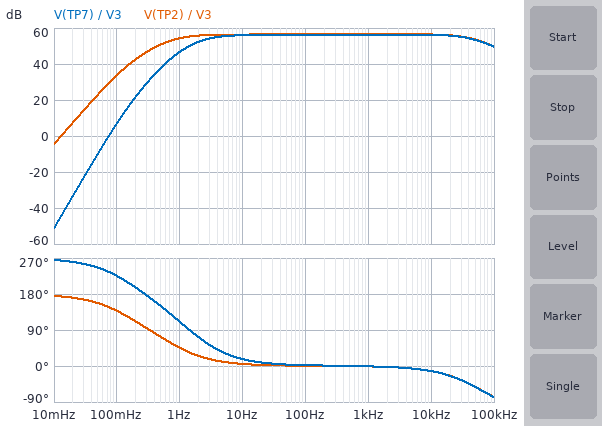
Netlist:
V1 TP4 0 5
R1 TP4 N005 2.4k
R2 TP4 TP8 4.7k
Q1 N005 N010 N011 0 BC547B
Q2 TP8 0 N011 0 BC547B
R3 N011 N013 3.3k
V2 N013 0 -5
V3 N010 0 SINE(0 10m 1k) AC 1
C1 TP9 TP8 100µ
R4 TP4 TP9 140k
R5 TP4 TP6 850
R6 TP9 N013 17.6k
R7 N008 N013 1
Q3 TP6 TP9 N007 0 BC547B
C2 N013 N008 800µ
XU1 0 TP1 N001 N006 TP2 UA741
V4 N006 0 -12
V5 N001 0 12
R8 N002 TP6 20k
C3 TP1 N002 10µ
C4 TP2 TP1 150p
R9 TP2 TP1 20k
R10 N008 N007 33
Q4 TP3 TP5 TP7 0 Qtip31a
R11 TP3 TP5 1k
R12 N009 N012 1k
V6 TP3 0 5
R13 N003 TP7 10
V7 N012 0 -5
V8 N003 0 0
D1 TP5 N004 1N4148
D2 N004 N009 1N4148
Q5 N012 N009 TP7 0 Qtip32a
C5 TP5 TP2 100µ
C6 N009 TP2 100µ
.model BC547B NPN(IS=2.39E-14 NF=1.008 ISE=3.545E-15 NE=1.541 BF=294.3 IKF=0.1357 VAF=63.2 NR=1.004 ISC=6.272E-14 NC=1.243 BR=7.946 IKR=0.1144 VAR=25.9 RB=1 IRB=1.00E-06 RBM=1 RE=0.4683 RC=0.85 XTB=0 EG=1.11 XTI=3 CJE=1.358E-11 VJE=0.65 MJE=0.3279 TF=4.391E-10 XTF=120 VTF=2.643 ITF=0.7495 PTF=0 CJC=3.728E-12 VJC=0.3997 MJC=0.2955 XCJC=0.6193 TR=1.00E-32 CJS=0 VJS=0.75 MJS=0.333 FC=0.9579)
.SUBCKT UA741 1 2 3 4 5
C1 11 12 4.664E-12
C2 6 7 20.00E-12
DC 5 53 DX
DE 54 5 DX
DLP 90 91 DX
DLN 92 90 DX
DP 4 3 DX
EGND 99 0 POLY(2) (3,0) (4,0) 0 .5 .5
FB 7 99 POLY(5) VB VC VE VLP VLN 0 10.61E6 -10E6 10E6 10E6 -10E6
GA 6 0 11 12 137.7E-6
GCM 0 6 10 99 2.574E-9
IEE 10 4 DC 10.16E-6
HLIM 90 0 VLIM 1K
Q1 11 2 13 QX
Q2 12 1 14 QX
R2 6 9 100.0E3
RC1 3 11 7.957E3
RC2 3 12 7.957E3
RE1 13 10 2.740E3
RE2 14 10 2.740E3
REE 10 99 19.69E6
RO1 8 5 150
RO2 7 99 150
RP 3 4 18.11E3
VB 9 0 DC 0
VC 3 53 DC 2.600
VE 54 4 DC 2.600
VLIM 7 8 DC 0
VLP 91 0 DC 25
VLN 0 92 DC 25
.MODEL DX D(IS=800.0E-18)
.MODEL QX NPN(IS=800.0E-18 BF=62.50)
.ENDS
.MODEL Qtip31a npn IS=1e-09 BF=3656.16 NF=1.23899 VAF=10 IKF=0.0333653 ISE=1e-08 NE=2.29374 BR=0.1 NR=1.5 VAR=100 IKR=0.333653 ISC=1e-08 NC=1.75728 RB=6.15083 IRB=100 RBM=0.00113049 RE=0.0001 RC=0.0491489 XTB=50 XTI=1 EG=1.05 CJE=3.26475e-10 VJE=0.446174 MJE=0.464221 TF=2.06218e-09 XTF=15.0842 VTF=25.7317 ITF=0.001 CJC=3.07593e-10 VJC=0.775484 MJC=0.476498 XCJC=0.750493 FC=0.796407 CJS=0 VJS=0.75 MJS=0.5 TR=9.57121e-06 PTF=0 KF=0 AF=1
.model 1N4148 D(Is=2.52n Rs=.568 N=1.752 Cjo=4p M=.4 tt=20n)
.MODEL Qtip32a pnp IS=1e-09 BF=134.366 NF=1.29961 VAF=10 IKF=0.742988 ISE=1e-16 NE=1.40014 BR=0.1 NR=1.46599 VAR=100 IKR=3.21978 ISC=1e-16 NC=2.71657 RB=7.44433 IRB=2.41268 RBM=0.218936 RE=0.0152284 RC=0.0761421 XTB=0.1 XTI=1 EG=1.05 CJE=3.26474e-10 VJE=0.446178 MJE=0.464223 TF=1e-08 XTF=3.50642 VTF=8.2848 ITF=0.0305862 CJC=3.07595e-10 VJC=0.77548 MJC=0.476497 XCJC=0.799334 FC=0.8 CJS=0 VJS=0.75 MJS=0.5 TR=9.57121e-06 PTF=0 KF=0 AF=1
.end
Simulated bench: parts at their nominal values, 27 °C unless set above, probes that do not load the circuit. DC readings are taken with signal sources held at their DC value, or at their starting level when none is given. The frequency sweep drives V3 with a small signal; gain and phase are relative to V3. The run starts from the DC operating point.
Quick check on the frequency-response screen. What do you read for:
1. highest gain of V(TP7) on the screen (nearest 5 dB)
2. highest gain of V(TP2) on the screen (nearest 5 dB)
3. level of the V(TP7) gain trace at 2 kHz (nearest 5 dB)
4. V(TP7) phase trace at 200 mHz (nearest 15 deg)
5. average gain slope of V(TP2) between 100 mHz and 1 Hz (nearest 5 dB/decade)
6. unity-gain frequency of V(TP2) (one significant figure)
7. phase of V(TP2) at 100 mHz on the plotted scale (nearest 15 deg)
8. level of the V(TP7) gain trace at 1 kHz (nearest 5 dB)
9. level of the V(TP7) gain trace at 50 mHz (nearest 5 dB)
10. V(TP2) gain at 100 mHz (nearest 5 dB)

55 dB
55 dB
55 dB
195 deg
20 dB/decade
10 mHz
135 deg
55 dB
-10 dB
35 dB
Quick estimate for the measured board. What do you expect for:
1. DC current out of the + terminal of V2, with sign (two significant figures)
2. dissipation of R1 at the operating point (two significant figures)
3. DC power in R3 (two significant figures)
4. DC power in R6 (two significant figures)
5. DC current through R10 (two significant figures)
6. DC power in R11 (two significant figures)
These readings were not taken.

-6.4 mA
1.1 mW
5.8 mW
41 µW
5.0 mA
18 mW
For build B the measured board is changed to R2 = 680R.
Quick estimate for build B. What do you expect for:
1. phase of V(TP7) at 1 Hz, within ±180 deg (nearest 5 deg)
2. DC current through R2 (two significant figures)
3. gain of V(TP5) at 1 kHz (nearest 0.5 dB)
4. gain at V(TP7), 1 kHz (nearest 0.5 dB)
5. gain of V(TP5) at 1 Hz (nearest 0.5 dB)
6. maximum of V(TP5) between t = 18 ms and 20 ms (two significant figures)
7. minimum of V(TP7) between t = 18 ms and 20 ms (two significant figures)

115 deg
670 µA
44.0 dB
43.5 dB
34.0 dB
2.3 V
-1.3 V
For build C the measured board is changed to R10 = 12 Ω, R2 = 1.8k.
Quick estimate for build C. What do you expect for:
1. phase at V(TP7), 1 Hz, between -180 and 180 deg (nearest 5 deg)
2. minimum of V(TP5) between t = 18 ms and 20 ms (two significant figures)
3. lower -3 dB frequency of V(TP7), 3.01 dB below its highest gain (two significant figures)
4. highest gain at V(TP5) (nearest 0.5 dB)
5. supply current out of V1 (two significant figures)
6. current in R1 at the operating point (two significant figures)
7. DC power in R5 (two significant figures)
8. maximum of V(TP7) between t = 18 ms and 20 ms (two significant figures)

120 deg
-4.2 V
2.6 Hz
56.5 dB
7.8 mA
660 µA
35 mW
4.4 V
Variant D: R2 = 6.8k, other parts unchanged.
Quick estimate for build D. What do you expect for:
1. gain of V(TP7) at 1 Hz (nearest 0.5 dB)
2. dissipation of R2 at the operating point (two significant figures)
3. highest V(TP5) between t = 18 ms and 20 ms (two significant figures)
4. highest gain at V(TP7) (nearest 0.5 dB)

48.5 dB
2.8 mW
5.6 V
58.0 dB
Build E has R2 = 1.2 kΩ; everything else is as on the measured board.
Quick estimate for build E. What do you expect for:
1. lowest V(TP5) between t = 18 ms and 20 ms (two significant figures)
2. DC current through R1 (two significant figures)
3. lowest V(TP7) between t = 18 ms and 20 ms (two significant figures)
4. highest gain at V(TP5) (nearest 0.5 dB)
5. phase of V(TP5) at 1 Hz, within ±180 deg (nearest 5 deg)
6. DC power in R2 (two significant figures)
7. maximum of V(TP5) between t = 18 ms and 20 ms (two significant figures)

-1.6 V
660 µA
-2.2 V
48.0 dB
115 deg
530 µW
3.3 V
